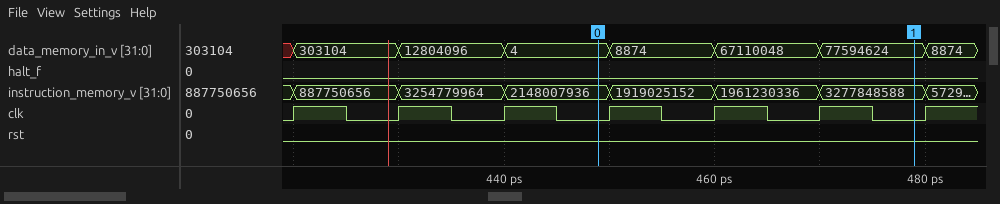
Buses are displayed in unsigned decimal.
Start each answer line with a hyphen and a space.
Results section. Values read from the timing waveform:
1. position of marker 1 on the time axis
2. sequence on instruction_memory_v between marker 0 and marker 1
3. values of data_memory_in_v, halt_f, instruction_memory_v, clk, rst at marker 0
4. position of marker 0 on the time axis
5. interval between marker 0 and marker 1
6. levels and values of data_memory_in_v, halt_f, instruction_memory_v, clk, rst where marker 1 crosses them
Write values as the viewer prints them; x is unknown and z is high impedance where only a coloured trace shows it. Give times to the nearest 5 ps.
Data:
- 480 ps
- 2148007936, 1919025152, 1961230336, 3277848588
- data_memory_in_v=4, halt_f=0, instruction_memory_v=2148007936, clk=0, rst=0
- 450 ps
- 30 ps
- data_memory_in_v=77594624, halt_f=0, instruction_memory_v=3277848588, clk=0, rst=0
